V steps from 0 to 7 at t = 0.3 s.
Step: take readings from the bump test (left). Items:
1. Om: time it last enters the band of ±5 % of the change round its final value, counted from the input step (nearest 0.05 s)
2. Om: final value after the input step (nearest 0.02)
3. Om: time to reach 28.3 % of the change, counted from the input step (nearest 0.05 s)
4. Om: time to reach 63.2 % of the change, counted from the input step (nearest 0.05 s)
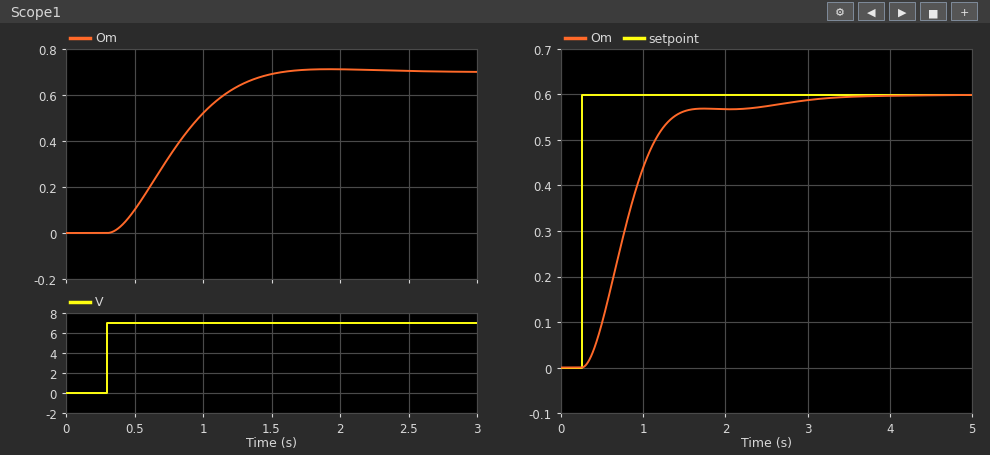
1.05 s
0.70
0.30 s
0.60 s
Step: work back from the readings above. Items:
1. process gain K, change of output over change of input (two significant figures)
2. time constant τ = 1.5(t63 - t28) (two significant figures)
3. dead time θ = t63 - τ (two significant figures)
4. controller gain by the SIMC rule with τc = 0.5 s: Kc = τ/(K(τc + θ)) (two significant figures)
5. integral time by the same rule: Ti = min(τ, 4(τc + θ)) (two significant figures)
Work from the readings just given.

0.10
0.45 s
0.15 s
6.9
0.45 s
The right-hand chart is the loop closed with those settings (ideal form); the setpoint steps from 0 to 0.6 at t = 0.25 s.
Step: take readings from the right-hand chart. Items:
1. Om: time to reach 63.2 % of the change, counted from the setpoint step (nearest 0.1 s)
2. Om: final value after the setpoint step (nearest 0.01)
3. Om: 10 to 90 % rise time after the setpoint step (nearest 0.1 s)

0.6 s
0.60
0.9 s
